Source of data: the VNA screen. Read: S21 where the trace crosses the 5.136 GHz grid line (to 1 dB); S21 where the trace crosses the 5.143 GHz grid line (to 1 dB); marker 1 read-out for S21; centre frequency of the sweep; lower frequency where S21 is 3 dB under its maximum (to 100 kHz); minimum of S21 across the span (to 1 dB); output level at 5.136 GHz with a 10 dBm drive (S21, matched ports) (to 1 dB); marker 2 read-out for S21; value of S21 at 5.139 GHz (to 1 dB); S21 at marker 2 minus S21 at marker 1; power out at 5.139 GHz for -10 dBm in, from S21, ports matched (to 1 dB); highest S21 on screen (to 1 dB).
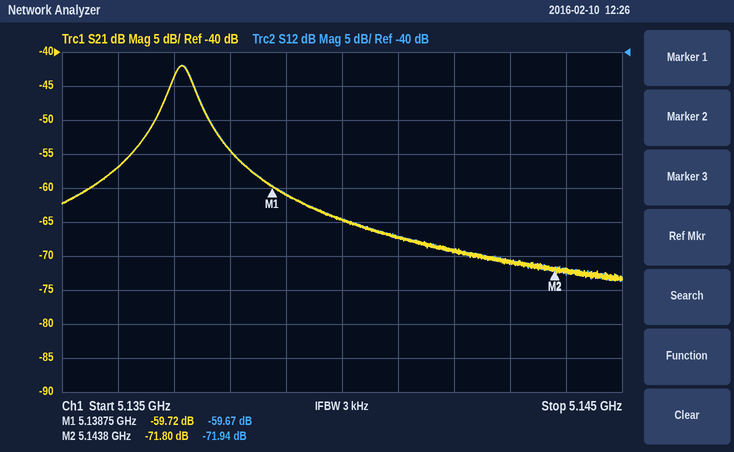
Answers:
-57 dB
-71 dB
-59.72 dB
5.14 GHz
5.1369 GHz
-74 dB
-47 dBm
-71.80 dB
-61 dB
-12.08 dB
-71 dBm
-42 dB
